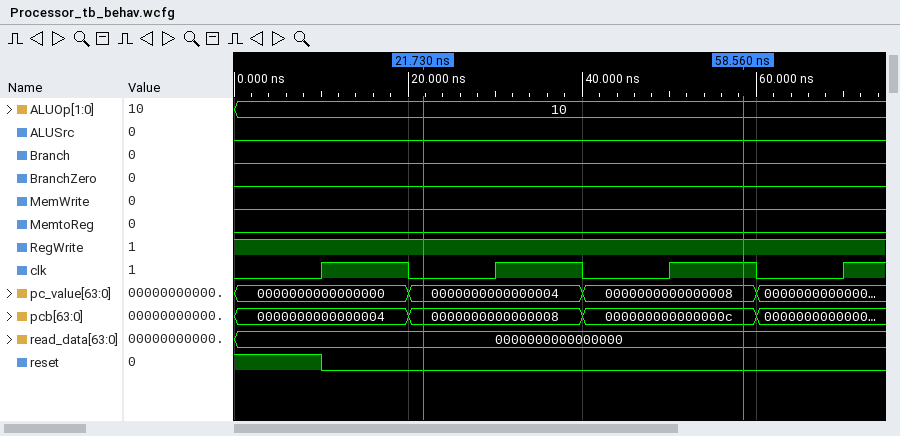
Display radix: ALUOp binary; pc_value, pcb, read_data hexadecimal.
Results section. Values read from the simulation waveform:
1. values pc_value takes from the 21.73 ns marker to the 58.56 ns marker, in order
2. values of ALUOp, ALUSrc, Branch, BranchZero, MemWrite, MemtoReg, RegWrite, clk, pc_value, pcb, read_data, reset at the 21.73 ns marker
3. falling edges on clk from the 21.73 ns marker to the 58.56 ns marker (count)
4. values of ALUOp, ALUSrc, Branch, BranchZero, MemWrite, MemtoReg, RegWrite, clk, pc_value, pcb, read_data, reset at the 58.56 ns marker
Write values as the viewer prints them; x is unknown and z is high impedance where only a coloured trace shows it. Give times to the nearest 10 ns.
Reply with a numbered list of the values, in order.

1. 0000000000000004, 0000000000000008
2. ALUOp=10, ALUSrc=0, Branch=0, BranchZero=0, MemWrite=0, MemtoReg=0, RegWrite=1, clk=0, pc_value=0000000000000004, pcb=0000000000000008, read_data=0000000000000000, reset=0
3. 1
4. ALUOp=10, ALUSrc=0, Branch=0, BranchZero=0, MemWrite=0, MemtoReg=0, RegWrite=1, clk=1, pc_value=0000000000000008, pcb=000000000000000c, read_data=0000000000000000, reset=0
